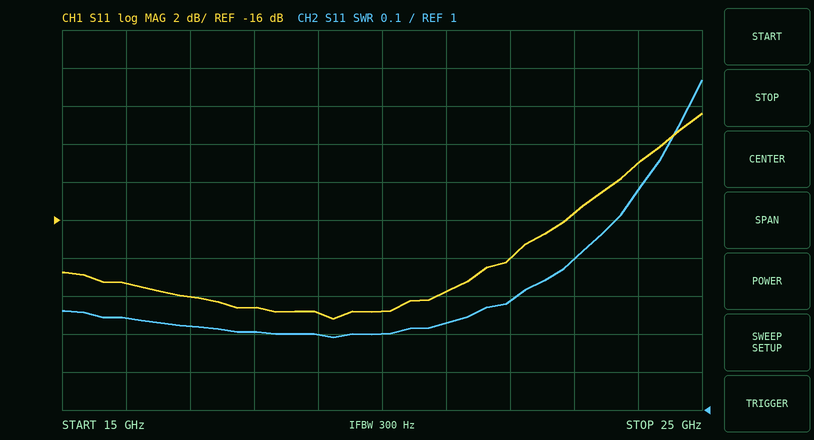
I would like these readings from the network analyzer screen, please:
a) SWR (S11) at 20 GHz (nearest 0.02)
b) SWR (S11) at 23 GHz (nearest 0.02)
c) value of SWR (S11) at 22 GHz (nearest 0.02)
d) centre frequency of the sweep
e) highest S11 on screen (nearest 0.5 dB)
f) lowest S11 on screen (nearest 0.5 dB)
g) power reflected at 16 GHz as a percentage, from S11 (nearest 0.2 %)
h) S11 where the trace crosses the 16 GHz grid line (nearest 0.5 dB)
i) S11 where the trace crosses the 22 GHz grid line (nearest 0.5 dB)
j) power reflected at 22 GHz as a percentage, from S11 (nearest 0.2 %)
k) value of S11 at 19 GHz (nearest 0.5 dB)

1.20
1.40
1.28
20 GHz
-10.5 dB
-21.0 dB
1.2 %
-19.5 dB
-18.0 dB
1.6 %
-21.0 dB
